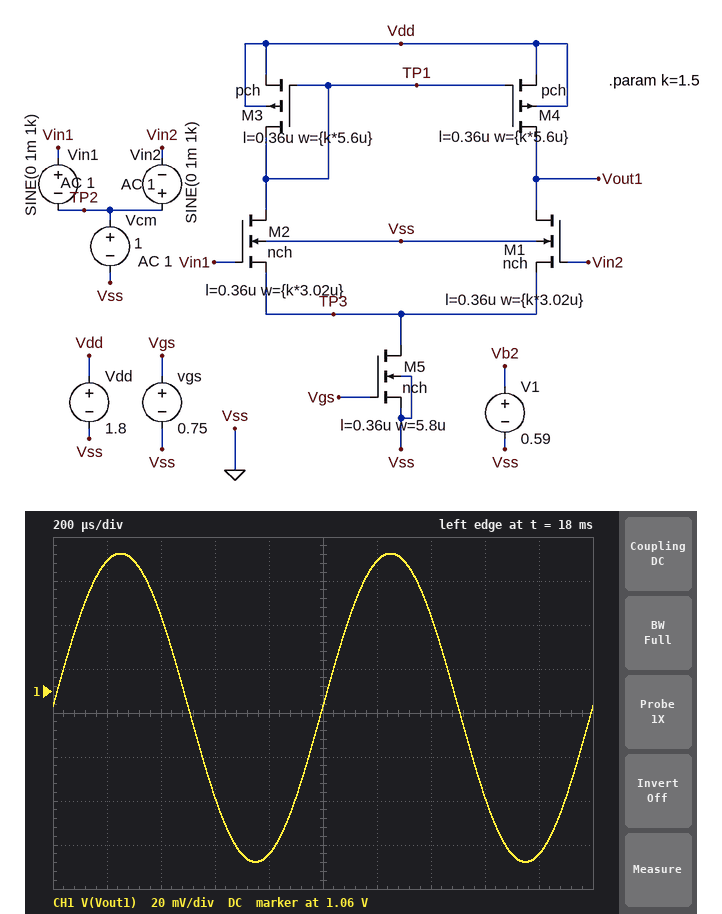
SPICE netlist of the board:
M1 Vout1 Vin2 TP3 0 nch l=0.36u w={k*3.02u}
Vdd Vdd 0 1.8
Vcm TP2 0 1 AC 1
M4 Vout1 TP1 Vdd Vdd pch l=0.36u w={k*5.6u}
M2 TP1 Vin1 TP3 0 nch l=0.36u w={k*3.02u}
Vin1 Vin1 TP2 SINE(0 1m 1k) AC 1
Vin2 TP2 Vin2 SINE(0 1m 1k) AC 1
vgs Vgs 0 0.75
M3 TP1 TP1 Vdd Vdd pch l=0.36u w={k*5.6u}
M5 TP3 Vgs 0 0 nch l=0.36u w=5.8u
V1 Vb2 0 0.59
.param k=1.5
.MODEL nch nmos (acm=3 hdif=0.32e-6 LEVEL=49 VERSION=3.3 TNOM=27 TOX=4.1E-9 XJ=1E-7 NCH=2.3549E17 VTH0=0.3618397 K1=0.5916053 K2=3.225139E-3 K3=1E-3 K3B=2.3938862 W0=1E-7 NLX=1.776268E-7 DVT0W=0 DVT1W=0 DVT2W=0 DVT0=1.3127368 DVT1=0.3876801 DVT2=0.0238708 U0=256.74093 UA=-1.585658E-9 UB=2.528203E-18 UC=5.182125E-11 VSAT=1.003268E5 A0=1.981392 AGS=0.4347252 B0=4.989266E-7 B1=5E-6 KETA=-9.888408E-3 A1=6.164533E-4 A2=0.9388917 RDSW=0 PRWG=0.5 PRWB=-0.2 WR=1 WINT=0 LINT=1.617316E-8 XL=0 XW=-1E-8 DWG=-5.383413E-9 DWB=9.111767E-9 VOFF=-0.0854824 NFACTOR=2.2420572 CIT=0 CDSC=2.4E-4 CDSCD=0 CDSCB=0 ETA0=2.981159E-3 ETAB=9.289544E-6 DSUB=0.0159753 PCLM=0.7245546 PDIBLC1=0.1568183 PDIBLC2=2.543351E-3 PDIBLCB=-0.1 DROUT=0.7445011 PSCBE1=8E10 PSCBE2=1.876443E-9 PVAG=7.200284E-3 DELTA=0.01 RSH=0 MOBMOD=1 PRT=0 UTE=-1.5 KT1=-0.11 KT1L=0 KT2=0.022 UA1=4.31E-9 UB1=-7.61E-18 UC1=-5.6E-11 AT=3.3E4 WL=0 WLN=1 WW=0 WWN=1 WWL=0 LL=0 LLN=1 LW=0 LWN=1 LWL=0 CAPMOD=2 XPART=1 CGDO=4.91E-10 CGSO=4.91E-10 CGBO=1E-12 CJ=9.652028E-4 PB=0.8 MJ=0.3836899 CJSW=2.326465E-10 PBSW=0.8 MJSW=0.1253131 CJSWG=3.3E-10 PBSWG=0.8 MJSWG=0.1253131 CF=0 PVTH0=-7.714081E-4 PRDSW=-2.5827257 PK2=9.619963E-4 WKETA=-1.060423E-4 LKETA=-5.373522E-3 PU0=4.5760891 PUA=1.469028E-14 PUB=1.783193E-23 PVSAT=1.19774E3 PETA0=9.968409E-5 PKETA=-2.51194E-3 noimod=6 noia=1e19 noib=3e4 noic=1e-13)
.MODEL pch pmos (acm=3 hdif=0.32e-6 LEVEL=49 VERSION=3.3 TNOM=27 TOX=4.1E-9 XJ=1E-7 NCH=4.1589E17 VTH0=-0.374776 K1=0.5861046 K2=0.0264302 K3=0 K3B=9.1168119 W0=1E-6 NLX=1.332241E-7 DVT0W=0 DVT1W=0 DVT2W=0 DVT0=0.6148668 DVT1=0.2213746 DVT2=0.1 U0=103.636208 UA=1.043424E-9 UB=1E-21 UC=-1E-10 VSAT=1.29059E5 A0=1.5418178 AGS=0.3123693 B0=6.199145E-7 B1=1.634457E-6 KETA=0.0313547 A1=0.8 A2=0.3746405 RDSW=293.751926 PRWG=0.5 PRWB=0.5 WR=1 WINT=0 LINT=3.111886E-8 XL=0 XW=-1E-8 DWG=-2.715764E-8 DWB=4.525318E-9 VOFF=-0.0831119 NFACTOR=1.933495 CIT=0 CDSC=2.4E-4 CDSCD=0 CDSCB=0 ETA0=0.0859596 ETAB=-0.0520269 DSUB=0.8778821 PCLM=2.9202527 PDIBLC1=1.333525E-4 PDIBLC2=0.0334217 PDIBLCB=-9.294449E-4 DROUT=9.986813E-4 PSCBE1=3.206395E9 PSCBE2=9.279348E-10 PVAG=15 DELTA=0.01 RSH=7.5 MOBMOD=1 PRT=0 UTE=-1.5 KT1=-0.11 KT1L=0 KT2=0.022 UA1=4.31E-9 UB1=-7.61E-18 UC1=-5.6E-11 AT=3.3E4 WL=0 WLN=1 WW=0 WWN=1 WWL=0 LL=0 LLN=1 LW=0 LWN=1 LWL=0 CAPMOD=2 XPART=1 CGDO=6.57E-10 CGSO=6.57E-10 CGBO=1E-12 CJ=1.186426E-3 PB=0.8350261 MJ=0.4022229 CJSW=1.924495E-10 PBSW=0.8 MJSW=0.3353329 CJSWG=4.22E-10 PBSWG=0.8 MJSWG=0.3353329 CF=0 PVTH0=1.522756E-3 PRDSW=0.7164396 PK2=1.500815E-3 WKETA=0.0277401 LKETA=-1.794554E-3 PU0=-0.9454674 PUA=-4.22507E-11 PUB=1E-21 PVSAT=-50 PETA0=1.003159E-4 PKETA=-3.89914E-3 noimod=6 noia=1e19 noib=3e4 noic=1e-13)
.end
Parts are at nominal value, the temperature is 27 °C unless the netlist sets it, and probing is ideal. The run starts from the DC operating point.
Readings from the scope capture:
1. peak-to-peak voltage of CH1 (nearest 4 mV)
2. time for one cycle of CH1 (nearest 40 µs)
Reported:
140 mV
1.00 ms
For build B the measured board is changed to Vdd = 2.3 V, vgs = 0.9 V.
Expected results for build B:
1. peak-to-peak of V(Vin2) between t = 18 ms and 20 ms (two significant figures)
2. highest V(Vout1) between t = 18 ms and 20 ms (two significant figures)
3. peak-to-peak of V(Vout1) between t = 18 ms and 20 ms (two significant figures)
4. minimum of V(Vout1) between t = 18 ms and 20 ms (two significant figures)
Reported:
2.0 mV
1.5 V
130 mV
1.4 V
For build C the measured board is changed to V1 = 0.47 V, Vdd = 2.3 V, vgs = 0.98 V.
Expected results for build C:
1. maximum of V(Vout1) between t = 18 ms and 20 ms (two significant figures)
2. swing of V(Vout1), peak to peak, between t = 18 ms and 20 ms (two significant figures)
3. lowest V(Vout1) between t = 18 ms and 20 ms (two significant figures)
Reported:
1.5 V
130 mV
1.3 V
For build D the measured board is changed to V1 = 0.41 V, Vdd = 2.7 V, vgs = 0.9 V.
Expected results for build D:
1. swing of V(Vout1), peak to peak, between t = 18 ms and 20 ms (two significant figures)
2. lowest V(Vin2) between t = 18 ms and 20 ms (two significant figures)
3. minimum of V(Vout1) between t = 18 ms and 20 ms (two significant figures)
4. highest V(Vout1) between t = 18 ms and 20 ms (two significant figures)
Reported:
130 mV
1.0 V
1.8 V
1.9 V
